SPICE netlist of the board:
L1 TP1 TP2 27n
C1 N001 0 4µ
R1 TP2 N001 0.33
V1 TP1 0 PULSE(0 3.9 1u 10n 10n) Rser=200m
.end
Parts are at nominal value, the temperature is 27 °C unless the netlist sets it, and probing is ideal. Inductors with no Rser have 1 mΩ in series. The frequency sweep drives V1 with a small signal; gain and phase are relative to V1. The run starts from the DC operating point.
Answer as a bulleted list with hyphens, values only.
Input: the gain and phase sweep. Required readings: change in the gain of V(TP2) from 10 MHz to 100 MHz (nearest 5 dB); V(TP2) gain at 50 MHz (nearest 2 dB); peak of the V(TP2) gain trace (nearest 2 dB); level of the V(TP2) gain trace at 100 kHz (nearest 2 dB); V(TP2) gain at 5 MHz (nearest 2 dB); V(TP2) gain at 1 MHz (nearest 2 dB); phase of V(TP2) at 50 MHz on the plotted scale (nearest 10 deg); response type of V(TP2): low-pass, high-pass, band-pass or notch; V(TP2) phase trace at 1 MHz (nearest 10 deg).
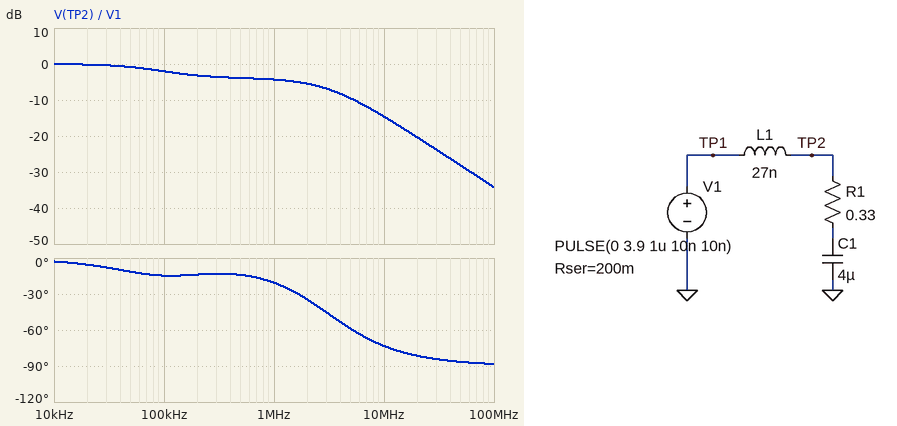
- -20 dB
- -28 dB
- 0 dB
- -2 dB
- -10 dB
- -4 dB
- -90 deg
- low-pass
- -20 deg
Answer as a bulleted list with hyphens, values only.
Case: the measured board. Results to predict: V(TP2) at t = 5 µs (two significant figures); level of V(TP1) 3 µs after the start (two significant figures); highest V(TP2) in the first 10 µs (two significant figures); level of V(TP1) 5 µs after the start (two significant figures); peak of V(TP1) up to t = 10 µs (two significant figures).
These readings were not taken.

- 3.7 V
- 3.3 V
- 3.9 V
- 3.7 V
- 3.9 V
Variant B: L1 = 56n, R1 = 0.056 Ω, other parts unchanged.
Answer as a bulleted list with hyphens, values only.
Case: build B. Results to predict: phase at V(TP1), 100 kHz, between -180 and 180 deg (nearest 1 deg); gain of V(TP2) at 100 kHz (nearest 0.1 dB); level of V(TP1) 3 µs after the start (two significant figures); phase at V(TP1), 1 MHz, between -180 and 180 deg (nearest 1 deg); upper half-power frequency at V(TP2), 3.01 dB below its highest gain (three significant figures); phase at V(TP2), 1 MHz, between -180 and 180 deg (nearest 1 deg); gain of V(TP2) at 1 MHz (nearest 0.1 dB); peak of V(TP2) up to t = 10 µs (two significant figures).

- -26 deg
- -0.9 dB
- 3.4 V
- 29 deg
- 207 kHz
- -86 deg
- -15.4 dB
- 3.9 V
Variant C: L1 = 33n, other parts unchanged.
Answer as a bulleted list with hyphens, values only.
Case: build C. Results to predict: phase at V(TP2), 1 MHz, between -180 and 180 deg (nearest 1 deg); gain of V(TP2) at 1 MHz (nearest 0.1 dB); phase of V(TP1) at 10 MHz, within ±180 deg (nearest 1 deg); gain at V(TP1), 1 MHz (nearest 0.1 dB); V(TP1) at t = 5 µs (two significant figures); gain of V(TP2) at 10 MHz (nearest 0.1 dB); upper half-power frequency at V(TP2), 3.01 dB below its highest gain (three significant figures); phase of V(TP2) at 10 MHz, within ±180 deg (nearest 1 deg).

- -24 deg
- -4.5 dB
- 5 deg
- -3.5 dB
- 3.7 V
- -16.2 dB
- 180 kHz
- -76 deg
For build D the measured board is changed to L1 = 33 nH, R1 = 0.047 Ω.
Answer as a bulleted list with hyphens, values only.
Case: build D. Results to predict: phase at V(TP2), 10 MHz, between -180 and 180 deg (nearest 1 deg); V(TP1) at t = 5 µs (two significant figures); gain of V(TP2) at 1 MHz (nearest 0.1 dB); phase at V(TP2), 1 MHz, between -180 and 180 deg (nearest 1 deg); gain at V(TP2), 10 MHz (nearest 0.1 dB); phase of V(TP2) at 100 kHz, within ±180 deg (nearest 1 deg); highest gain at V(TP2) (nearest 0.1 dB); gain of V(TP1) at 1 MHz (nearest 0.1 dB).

- -88 deg
- 3.9 V
- -13.7 dB
- -74 deg
- -32.9 dB
- -27 deg
- 0 dB
- -4.7 dB
